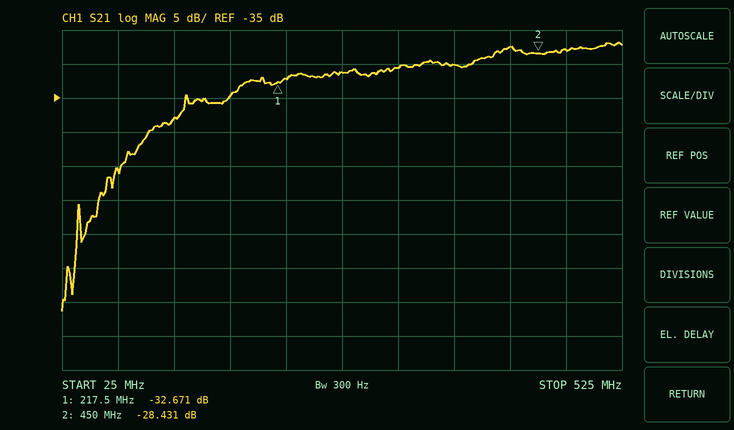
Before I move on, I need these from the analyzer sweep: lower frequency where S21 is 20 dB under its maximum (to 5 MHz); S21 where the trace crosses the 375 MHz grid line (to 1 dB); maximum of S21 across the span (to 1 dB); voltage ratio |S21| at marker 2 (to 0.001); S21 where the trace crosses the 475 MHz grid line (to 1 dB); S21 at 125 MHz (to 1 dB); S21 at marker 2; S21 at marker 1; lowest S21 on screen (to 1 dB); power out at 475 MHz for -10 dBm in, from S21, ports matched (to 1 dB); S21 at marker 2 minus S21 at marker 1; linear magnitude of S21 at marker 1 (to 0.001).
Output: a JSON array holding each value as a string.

["70 MHz", "-30 dB", "-27 dB", "0.038", "-28 dB", "-38 dB", "-28.431 dB", "-32.671 dB", "-66 dB", "-38 dBm", "4.240 dB", "0.023"]
